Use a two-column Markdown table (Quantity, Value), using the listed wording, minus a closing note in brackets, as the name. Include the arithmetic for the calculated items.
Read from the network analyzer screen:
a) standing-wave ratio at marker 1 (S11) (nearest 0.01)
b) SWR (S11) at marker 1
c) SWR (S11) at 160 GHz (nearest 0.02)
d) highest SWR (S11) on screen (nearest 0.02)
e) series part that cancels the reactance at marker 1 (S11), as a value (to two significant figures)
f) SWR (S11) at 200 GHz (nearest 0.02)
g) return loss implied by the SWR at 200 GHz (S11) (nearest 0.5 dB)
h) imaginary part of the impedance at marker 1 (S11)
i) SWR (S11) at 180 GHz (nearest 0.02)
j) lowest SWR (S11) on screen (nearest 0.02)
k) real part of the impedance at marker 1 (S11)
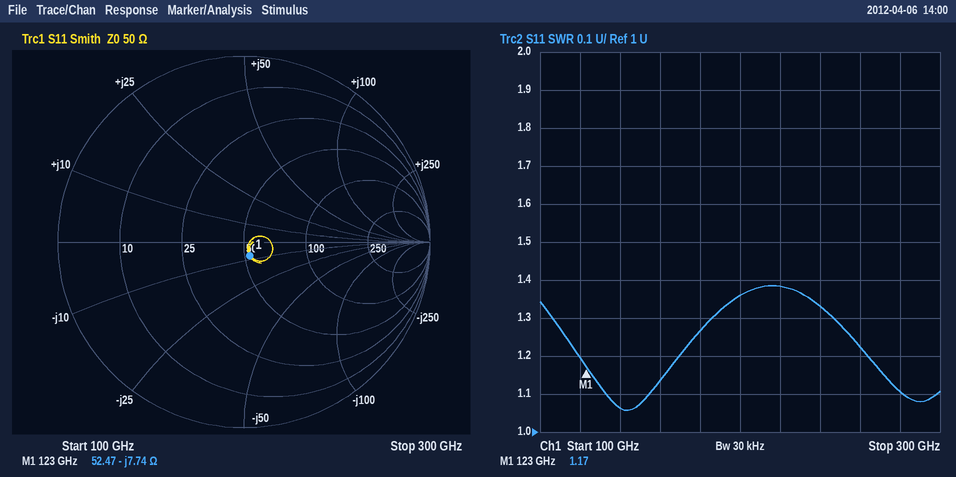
| Quantity | Value |
|---|---|
| standing-wave ratio at marker 1 (S11) | 1.17 |
| SWR (S11) at marker 1 | 1.17 |
| SWR (S11) at 160 GHz | 1.14 |
| highest SWR (S11) on screen | 1.38 |
| series part that cancels the reactance at marker 1 (S11), as a value | L = 7.74 Ω/(2π × 123 GHz) ≈ 10 pH |
| SWR (S11) at 200 GHz | 1.36 |
| return loss implied by the SWR at 200 GHz (S11) | −20 log10((1.36 − 1)/(1.36 + 1)) ≈ 16.3 dB, so 16.5 dB to the nearest 0.5 dB |
| imaginary part of the impedance at marker 1 | -7.74 Ω |
| SWR (S11) at 180 GHz | 1.26 |
| lowest SWR (S11) on screen | 1.06 |
| real part of the impedance at marker 1 | 52.47 Ω |
